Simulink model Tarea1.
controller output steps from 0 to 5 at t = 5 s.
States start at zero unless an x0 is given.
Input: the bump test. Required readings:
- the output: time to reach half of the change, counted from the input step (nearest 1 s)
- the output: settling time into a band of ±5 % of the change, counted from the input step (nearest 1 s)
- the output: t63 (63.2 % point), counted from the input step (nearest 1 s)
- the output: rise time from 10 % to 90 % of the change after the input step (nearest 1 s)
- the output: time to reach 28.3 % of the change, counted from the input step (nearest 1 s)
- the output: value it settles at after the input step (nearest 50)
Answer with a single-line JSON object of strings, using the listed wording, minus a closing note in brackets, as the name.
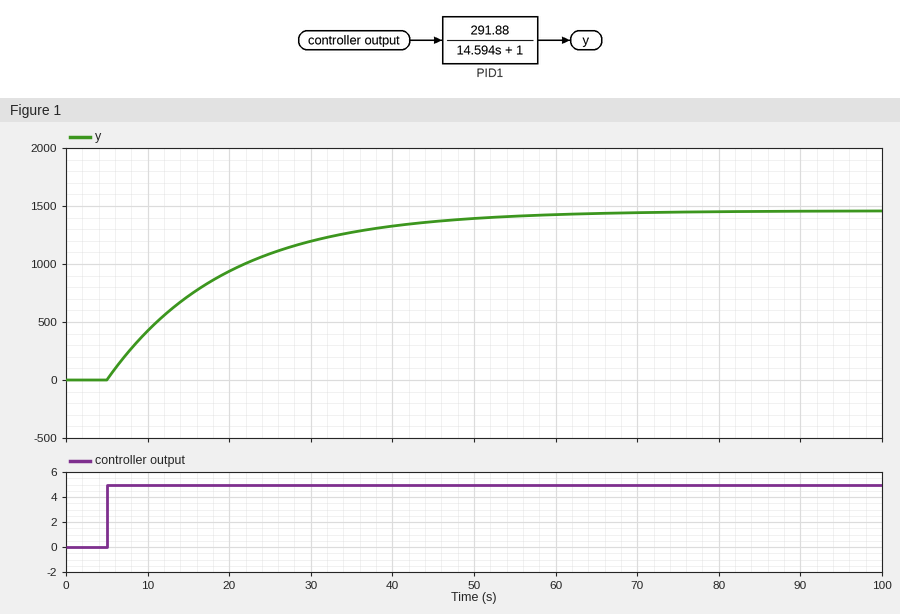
{"the output: time to reach half of the change, counted from the input step": "10 s", "the output: settling time into a band of ±5 % of the change, counted from the input step": "44 s", "the output: t63 (63.2 % point), counted from the input step": "15 s", "the output: rise time from 10 % to 90 % of the change after the input step": "32 s", "the output: time to reach 28.3 % of the change, counted from the input step": "5 s", "the output: value it settles at after the input step": "1450"}
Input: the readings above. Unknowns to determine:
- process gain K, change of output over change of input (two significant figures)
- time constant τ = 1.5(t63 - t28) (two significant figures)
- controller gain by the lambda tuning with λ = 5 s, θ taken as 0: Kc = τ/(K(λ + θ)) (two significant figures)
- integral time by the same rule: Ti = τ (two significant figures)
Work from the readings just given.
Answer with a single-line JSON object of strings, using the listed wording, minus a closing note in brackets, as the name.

{"process gain K, change of output over change of input": "290", "time constant τ = 1.5(t63 - t28)": "15 s", "controller gain by the lambda tuning with λ = 5 s, θ taken as 0: Kc = τ/(K(λ + θ))": "0.010", "integral time by the same rule: Ti = τ": "15 s"}
